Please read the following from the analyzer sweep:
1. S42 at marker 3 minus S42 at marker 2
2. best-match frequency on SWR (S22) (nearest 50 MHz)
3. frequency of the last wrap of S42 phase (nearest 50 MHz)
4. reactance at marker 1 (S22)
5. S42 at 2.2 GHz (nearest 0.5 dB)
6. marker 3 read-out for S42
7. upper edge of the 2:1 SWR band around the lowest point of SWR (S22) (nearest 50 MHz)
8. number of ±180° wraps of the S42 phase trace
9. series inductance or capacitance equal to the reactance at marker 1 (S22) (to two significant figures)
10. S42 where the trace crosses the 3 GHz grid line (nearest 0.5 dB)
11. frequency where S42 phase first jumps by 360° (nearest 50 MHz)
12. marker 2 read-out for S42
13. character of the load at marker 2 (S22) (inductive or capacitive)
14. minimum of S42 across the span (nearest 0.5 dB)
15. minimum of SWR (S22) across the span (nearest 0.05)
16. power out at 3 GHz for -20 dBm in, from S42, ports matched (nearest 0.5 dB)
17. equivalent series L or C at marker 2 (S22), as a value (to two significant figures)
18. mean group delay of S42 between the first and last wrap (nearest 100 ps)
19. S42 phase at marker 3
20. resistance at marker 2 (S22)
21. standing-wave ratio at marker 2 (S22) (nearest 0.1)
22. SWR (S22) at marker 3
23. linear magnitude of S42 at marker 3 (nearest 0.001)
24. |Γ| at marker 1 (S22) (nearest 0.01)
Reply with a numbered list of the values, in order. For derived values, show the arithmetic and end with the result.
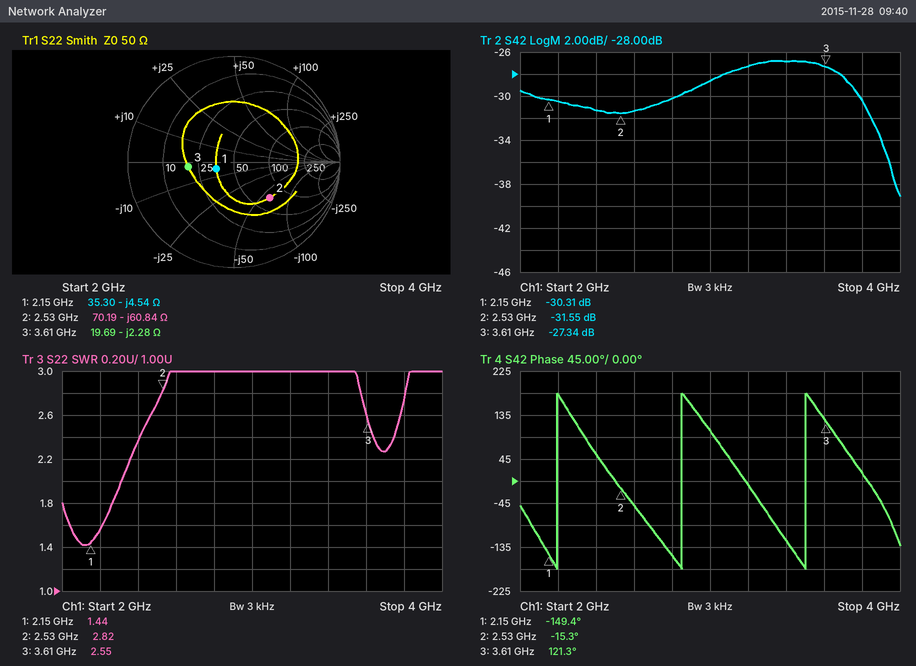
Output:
1. -27.34 − (-31.55) = 4.21 dB
2. 2.10 GHz
3. 3.50 GHz
4. -4.54 Ω
5. -30.5 dB
6. -27.34 dB
7. 2.30 GHz
8. 3
9. C = 1/(2π × 2.15 GHz × 4.54 Ω) ≈ 16 pF
10. -28.5 dB
11. 2.20 GHz
12. -31.55 dB
13. capacitive
14. -39.0 dB
15. 1.40
16. -20 dBm + (-28.5 dB) = -48.5 dBm
17. C = 1/(2π × 2.53 GHz × 60.84 Ω) ≈ 1.0 pF
18. 2 cycles / (3.50 GHz − 2.20 GHz) ≈ 1.5 ns
19. 121.3°
20. 70.19 Ω
21. 2.8
22. 2.55
23. 10^(-27.34/20) ≈ 0.043
24. 0.18
